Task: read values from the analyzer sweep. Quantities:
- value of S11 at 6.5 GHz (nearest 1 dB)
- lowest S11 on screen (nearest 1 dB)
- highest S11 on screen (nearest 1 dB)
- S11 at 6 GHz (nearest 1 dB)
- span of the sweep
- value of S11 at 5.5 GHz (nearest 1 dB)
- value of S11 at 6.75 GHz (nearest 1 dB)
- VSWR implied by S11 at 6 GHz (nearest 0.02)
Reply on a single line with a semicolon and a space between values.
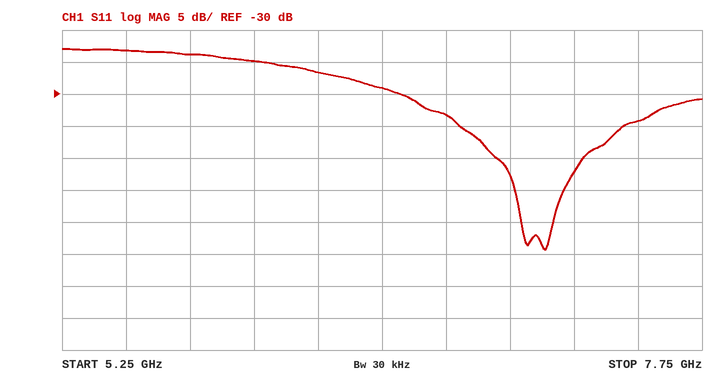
-29 dB; -54 dB; -23 dB; -25 dB; 2.5 GHz; -23 dB; -33 dB; 1.12
